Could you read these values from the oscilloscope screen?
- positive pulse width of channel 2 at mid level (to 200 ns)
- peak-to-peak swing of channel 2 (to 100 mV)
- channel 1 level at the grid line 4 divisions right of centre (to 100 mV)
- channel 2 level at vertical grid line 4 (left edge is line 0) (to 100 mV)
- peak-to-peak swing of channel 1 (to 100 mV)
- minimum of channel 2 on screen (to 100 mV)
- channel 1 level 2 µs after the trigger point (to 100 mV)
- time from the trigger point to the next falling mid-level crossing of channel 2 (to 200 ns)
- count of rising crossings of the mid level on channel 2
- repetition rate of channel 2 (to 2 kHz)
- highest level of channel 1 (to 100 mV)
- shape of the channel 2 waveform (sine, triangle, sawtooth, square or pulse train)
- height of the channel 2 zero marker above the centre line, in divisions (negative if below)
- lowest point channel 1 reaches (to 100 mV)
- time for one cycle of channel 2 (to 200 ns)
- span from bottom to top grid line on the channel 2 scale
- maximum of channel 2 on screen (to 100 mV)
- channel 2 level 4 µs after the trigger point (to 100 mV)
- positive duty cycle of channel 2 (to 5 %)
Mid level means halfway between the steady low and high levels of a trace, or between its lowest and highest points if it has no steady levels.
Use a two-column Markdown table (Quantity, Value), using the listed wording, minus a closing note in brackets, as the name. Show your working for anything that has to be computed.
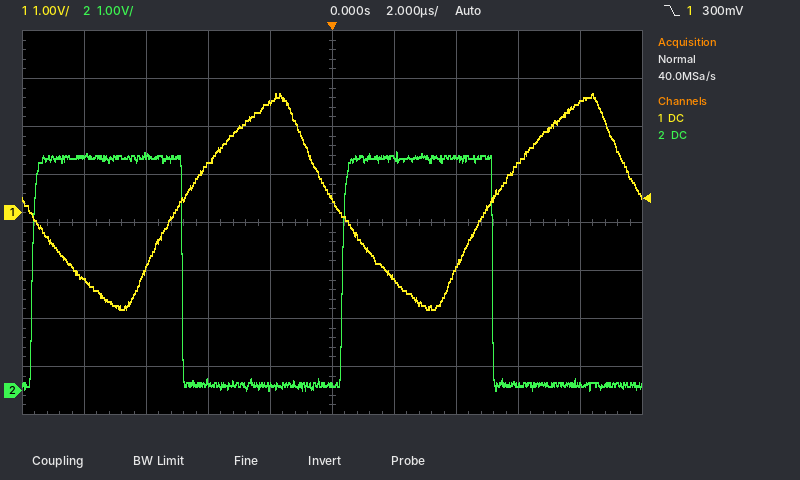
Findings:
| Quantity | Value |
|---|---|
| positive pulse width of channel 2 at mid level | 4.8 µs |
| peak-to-peak swing of channel 2 | 5.0 V − (0.0 V) = 5.0 V |
| channel 1 level at the grid line 4 divisions right of centre | 2.3 V |
| channel 2 level at vertical grid line 4 (left edge is line 0) | 100 mV |
| peak-to-peak swing of channel 1 | 2.5 V − (-2.0 V) = 4.5 V |
| minimum of channel 2 on screen | 0.0 V |
| channel 1 level 2 µs after the trigger point | -1.4 V |
| time from the trigger point to the next falling mid-level crossing of channel 2 | 5.2 µs |
| count of rising crossings of the mid level on channel 2 | 2 |
| repetition rate of channel 2 | 1 / 10.0 µs ≈ 100 kHz |
| highest level of channel 1 | 2.5 V |
| shape of the channel 2 waveform | square |
| height of the channel 2 zero marker above the centre line, in divisions | -3.5 div |
| lowest point channel 1 reaches | -2.0 V |
| time for one cycle of channel 2 | 10.0 µs |
| span from bottom to top grid line on the channel 2 scale | 8 V |
| maximum of channel 2 on screen | 5.0 V |
| channel 2 level 4 µs after the trigger point | 4.9 V |
| positive duty cycle of channel 2 | 4.8 µs / 10.0 µs ≈ 48.0 %, so 50 % to the nearest 5 % |
